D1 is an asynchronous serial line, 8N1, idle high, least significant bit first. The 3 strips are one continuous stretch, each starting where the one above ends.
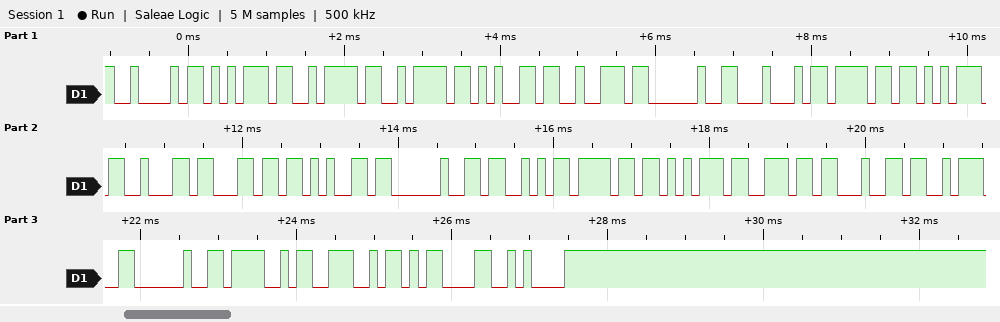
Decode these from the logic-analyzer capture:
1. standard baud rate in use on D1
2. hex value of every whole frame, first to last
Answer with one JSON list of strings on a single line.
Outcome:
["9600 baud", "42 75 7A 7A 65 72 20 44 6F 75 62 6C 65 20 53 6F 75 6E 64 3A 20 4F 4E 0D 0A"]
